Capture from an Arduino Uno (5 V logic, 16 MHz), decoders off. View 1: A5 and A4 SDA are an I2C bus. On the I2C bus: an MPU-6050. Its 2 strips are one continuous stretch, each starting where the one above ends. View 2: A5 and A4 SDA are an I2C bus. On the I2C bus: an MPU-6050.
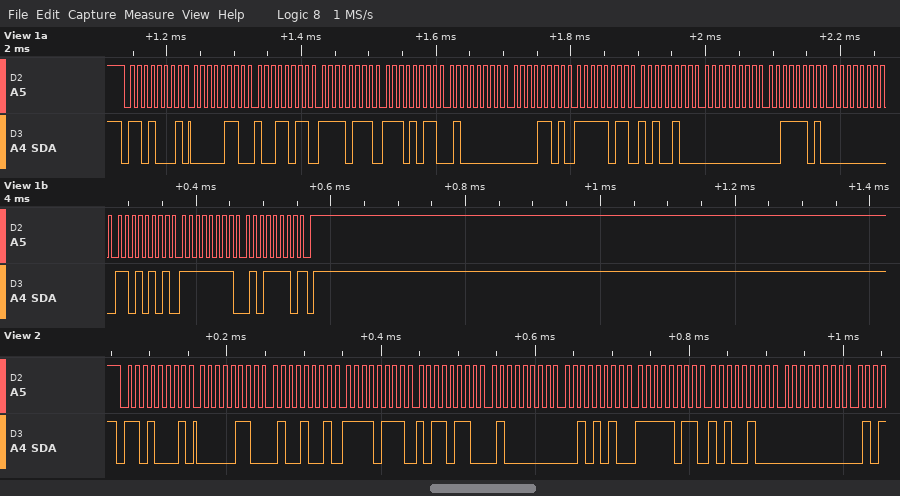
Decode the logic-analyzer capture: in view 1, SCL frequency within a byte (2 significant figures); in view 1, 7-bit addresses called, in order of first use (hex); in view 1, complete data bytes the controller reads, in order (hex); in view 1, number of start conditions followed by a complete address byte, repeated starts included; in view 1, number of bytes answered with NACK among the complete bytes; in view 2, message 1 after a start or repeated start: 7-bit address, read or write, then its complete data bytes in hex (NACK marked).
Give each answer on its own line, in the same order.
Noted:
100 kHz
0x68
06 9B F7 EB 40 0D FB A4 00 3D 00 D5 FF 5E
1
1
0x68 read: 06 49 F7 B6 40 2A FB A4 00
